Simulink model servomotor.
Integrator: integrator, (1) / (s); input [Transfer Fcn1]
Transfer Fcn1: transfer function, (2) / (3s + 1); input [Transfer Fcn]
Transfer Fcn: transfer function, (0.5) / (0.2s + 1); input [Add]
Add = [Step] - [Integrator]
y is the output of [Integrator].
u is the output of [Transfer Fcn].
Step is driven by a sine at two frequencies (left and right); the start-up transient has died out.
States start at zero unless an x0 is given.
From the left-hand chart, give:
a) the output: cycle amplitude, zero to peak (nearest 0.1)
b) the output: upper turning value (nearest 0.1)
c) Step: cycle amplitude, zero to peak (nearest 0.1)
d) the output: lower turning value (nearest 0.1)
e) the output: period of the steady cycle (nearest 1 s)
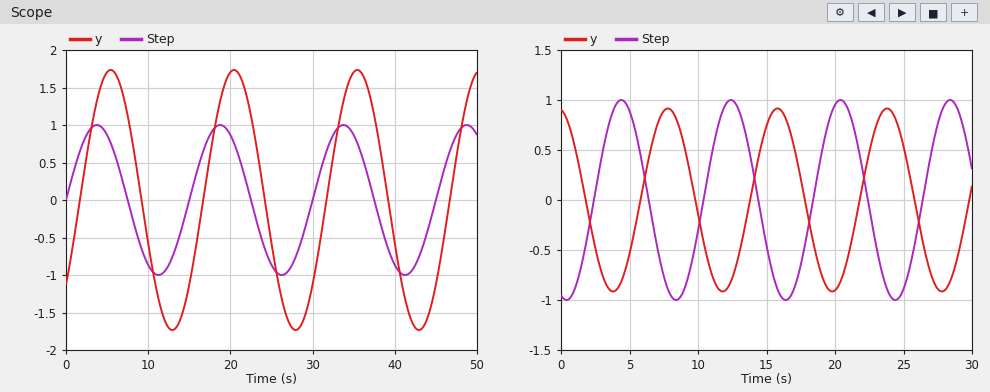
1.7
1.7
1.0
-1.7
15 s
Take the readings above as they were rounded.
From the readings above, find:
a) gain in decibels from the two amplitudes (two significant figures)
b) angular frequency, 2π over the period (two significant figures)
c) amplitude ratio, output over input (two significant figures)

4.6 dB
0.42 rad/s
1.7
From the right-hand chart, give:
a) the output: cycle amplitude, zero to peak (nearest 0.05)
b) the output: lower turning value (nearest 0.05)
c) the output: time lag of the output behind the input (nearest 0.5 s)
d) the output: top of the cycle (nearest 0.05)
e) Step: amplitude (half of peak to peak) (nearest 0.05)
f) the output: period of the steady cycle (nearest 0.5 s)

0.90
-0.90
3.5 s
0.90
1.00
8.0 s
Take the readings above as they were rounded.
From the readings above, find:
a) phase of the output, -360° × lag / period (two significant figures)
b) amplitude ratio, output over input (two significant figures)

-160°
0.90
